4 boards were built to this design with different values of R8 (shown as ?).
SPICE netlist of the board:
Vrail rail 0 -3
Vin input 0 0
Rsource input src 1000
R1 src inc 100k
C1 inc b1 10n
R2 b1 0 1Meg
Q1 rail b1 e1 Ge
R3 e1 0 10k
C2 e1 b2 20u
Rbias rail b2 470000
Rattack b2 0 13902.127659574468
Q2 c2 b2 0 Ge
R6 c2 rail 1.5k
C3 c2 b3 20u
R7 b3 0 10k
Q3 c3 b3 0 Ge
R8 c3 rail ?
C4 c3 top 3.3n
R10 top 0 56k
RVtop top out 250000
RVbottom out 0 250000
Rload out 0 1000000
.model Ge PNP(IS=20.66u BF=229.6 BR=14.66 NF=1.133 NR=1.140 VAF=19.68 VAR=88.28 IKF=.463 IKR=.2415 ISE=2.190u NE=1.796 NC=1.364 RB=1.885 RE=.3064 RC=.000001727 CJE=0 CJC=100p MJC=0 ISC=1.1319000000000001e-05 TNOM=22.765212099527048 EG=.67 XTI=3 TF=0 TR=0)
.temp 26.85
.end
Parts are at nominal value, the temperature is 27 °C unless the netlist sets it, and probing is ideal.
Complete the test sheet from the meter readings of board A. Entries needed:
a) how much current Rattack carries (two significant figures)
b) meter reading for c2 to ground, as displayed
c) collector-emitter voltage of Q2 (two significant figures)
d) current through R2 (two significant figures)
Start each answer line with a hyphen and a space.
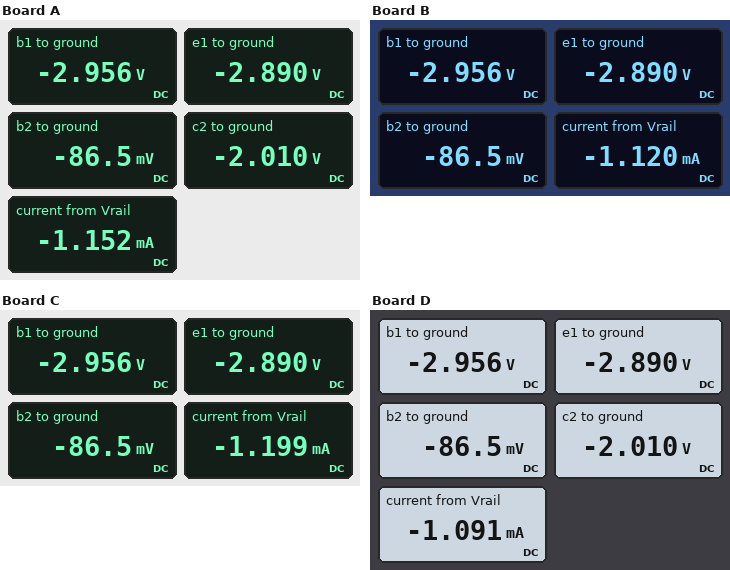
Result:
- 6.2 µA
- -2.010 V
- -2.0 V
- 3.0 µA
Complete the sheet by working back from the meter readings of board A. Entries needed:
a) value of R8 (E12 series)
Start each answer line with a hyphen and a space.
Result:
- 15 kΩ
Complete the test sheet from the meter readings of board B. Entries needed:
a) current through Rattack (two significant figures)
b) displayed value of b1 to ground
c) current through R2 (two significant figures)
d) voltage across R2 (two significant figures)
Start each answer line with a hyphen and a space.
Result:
- 6.2 µA
- -2.956 V
- 3.0 µA
- 3.0 V
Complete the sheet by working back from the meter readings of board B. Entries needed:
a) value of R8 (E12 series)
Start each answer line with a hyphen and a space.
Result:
- 18 kΩ
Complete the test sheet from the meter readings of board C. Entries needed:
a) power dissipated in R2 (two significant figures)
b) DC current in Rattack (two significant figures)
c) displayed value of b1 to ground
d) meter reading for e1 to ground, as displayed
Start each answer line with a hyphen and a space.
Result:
- 8.7 µW
- 6.2 µA
- -2.956 V
- -2.890 V
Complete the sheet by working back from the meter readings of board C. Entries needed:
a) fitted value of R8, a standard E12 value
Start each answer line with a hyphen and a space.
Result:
- 12 kΩ
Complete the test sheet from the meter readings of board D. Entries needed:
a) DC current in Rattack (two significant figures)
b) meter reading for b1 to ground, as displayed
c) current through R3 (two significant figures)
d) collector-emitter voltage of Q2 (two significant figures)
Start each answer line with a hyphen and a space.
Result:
- 6.2 µA
- -2.956 V
- 290 µA
- -2.0 V
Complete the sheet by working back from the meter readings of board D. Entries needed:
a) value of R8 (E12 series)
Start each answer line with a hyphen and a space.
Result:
- 22 kΩ
